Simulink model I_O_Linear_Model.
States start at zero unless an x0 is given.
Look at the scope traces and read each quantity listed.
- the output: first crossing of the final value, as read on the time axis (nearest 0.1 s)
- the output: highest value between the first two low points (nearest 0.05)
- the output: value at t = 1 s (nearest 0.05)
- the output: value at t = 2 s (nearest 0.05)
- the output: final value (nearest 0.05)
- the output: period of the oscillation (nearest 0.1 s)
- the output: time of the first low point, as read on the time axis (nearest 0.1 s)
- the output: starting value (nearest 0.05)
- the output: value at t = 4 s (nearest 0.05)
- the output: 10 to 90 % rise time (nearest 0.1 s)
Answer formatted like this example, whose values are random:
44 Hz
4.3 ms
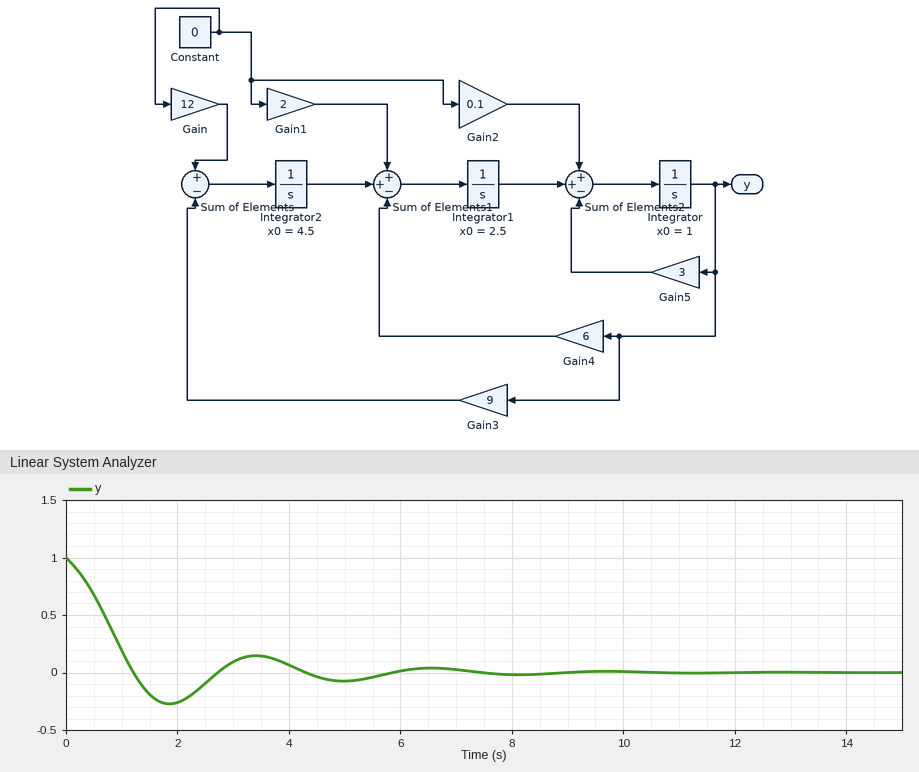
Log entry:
1.2 s
0.15
0.20
-0.25
0.00
3.1 s
1.9 s
1.00
0.05
0.9 s
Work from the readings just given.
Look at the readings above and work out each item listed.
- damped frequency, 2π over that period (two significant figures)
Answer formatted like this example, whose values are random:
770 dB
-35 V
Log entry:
2.0 rad/s
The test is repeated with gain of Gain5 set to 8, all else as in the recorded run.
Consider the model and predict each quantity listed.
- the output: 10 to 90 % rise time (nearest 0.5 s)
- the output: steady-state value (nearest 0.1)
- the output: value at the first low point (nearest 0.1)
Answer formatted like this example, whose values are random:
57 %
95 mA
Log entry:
2.0 s
0.0
-0.1
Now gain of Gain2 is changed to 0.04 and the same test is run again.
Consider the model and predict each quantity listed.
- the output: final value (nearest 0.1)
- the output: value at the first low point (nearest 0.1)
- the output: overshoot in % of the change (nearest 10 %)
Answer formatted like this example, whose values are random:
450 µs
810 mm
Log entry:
0.0
-0.3
30 %
